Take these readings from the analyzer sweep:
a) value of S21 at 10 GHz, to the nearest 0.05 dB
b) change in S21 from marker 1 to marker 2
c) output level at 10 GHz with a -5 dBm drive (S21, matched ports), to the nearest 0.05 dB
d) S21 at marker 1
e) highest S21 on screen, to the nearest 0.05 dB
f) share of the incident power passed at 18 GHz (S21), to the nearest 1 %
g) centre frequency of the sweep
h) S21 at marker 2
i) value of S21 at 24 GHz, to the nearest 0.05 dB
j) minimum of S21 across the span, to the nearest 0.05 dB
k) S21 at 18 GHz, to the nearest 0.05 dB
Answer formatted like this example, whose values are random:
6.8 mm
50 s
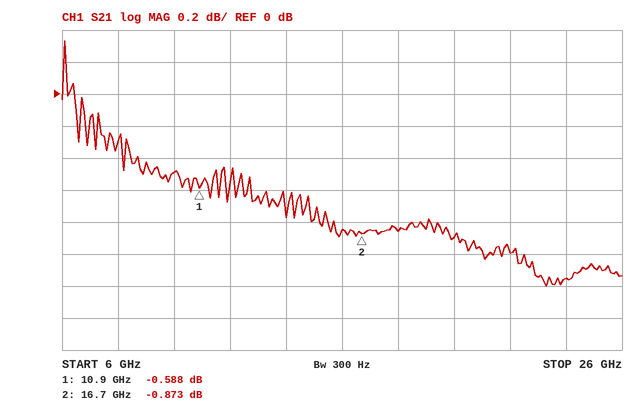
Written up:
-0.50 dB
-0.285 dB
-5.50 dBm
-0.588 dB
0.35 dB
82 %
16 GHz
-0.873 dB
-1.15 dB
-1.20 dB
-0.85 dB
